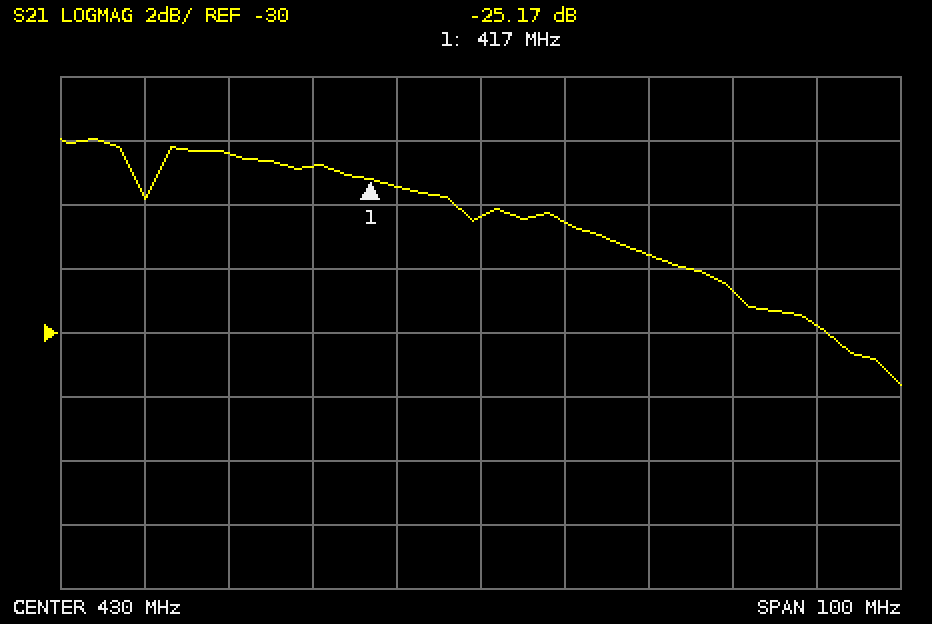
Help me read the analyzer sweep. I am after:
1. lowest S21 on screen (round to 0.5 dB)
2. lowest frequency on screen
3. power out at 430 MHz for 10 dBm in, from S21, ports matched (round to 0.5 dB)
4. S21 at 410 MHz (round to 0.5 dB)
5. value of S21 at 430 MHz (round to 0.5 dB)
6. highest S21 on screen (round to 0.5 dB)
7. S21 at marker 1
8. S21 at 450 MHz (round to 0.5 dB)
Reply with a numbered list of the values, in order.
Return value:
1. -31.5 dB
2. 380 MHz
3. -16.5 dBm
4. -25.0 dB
5. -26.5 dB
6. -24.0 dB
7. -25.17 dB
8. -27.5 dB
